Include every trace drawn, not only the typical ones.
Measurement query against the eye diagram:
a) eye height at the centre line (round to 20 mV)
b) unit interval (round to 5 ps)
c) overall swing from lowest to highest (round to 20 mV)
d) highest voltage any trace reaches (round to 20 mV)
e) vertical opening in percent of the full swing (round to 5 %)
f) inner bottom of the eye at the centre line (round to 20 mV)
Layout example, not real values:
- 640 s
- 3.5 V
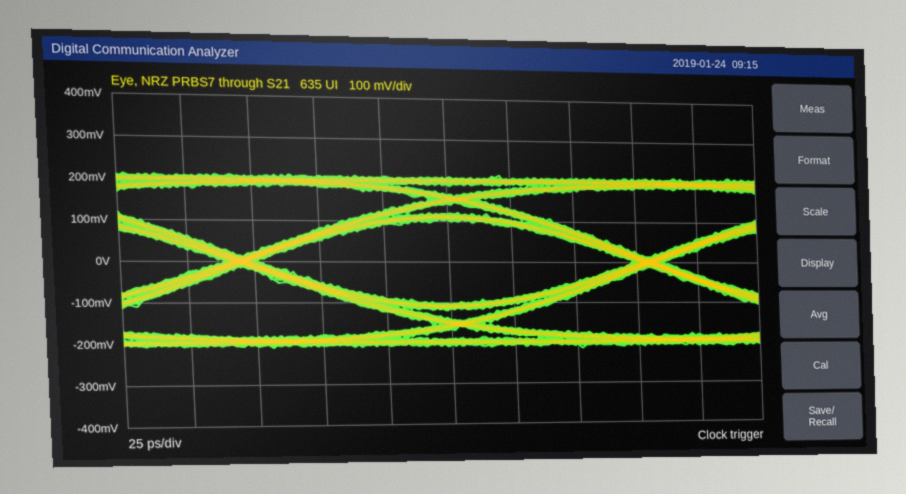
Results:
- 200 mV
- 160 ps
- 420 mV
- 220 mV
- 50 %
- -100 mV
